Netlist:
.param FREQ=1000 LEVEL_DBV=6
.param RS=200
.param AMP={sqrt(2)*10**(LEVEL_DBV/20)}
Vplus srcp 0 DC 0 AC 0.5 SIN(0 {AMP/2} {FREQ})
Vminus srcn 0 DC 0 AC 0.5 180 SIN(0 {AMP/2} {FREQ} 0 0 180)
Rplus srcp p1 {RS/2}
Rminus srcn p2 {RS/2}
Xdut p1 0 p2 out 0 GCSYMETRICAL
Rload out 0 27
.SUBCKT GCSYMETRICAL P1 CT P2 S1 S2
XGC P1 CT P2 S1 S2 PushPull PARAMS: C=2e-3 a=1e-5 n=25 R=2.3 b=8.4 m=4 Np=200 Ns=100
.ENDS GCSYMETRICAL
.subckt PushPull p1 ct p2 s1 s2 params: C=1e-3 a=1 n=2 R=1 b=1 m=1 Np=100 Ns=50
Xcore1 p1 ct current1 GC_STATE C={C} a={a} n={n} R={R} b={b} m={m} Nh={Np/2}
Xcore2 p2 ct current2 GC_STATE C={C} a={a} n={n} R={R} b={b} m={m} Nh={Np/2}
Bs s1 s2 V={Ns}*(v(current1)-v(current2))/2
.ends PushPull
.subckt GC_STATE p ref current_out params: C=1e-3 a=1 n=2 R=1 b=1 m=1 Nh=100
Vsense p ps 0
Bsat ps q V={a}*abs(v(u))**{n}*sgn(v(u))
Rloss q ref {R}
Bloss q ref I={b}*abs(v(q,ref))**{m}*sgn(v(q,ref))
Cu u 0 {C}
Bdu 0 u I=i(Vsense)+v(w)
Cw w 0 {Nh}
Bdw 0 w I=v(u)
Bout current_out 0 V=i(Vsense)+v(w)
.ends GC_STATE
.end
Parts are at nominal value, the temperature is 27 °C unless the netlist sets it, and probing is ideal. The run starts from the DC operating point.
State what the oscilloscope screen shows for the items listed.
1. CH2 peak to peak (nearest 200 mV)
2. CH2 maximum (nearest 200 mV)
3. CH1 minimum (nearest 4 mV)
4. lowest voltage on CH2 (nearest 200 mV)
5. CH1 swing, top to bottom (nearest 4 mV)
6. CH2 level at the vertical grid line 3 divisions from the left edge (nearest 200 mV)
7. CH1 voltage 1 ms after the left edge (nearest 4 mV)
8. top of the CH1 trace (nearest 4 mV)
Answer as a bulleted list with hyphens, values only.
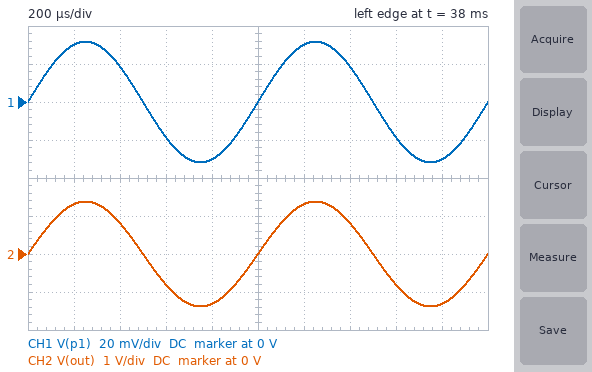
- 2.8 V
- 1.4 V
- -32 mV
- -1.4 V
- 64 mV
- -800 mV
- 0 V
- 32 mV
